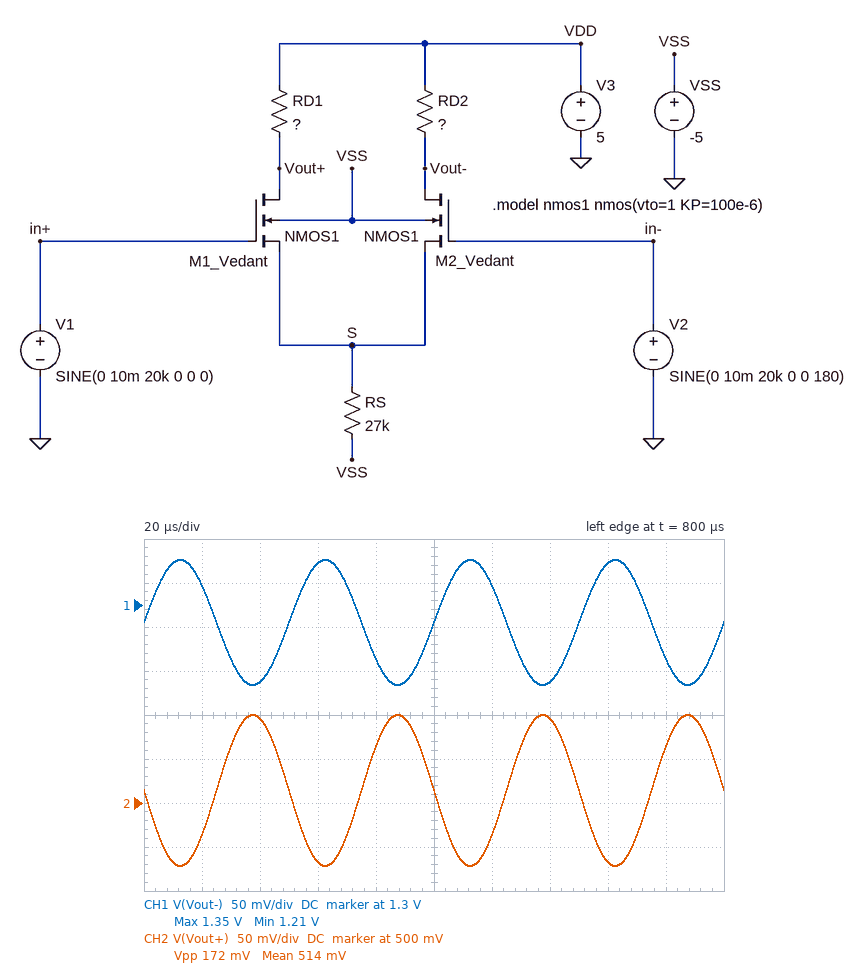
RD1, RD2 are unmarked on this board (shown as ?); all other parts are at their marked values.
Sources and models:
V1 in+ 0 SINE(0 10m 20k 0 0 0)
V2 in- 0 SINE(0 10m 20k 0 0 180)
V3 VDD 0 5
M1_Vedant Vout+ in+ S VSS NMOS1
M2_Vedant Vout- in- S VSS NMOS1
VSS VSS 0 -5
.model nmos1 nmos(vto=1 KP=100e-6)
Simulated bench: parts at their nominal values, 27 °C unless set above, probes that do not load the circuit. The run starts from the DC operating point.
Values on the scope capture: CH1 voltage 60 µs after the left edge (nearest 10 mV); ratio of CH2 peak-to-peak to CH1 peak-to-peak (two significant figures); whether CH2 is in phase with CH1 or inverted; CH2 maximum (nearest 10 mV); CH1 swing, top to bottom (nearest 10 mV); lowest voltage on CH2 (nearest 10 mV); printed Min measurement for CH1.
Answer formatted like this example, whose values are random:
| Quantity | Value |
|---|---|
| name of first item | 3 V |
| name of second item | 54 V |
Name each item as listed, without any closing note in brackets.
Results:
| Quantity | Value |
|---|---|
| CH1 voltage 60 µs after the left edge | 1.35 V |
| ratio of CH2 peak-to-peak to CH1 peak-to-peak | 1.2 |
| whether CH2 is in phase with CH1 or inverted | inverted |
| CH2 maximum | 600 mV |
| CH1 swing, top to bottom | 140 mV |
| lowest voltage on CH2 | 430 mV |
| printed Min measurement for CH1 | 1.21 V |
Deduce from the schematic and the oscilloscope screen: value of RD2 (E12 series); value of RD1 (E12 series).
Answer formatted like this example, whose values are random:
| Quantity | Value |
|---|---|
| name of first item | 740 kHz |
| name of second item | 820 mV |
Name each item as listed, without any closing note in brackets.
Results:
| Quantity | Value |
|---|---|
| value of RD2 | 68 kΩ |
| value of RD1 | 82 kΩ |
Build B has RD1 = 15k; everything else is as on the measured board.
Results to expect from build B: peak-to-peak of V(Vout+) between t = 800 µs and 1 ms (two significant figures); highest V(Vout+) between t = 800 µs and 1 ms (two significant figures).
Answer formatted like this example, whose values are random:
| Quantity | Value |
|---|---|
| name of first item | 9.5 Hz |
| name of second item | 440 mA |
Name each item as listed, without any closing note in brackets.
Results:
| Quantity | Value |
|---|---|
| peak-to-peak of V(Vout+) between t = 800 µs and 1 ms | 31 mV |
| highest V(Vout+) between t = 800 µs and 1 ms | 4.2 V |
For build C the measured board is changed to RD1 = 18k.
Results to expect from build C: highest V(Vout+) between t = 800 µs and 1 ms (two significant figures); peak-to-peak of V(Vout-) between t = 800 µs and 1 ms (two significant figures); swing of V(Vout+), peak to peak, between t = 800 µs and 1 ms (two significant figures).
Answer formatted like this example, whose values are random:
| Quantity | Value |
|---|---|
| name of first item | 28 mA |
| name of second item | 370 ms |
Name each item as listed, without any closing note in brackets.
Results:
| Quantity | Value |
|---|---|
| highest V(Vout+) between t = 800 µs and 1 ms | 4.0 V |
| peak-to-peak of V(Vout-) between t = 800 µs and 1 ms | 140 mV |
| swing of V(Vout+), peak to peak, between t = 800 µs and 1 ms | 38 mV |
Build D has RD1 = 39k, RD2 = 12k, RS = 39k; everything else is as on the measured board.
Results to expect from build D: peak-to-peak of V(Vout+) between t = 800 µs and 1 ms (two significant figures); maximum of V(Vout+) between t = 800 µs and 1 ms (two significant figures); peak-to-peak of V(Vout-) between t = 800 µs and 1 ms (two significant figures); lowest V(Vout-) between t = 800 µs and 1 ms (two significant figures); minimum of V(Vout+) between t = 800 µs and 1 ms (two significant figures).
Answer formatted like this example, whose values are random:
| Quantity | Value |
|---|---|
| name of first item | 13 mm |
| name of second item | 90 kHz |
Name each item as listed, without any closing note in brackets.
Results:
| Quantity | Value |
|---|---|
| peak-to-peak of V(Vout+) between t = 800 µs and 1 ms | 70 mV |
| maximum of V(Vout+) between t = 800 µs and 1 ms | 3.5 V |
| peak-to-peak of V(Vout-) between t = 800 µs and 1 ms | 21 mV |
| lowest V(Vout-) between t = 800 µs and 1 ms | 4.5 V |
| minimum of V(Vout+) between t = 800 µs and 1 ms | 3.4 V |
